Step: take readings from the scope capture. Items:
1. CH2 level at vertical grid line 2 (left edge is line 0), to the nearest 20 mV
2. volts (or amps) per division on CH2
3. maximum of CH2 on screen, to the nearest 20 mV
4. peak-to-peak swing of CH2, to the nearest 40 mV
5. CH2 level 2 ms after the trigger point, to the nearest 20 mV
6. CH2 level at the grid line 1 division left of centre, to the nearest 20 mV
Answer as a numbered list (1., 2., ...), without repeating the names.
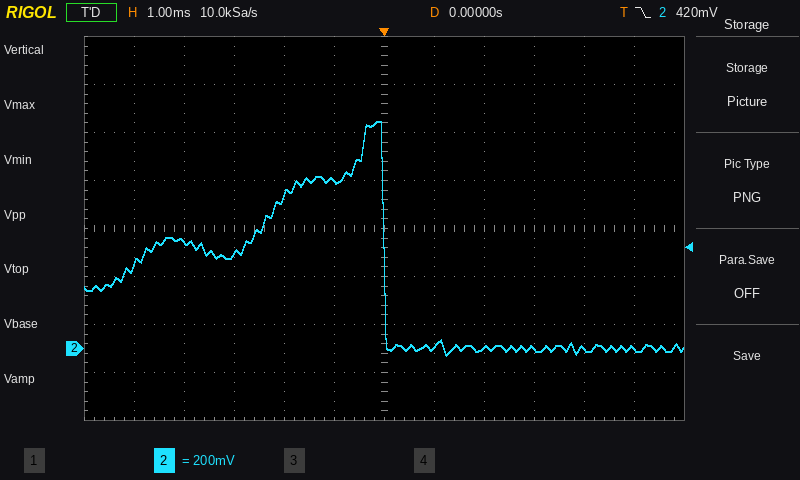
1. 440 mV
2. 200 mV
3. 940 mV
4. 960 mV
5. 0 mV
6. 700 mV
